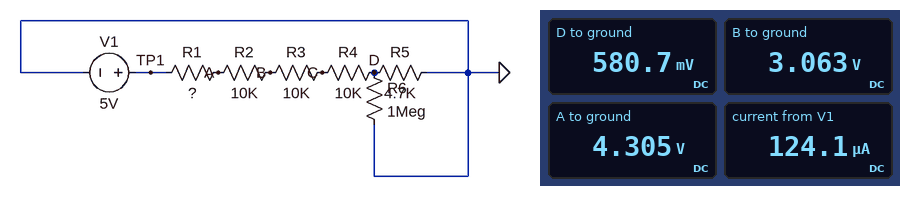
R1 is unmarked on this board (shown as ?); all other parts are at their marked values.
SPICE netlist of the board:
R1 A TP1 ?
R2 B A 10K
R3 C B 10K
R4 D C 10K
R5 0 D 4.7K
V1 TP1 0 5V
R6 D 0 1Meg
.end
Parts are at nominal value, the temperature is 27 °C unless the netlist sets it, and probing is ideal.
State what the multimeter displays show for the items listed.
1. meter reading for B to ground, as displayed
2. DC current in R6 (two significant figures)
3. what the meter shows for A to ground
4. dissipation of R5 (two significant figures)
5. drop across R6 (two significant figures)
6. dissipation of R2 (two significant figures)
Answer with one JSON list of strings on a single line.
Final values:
["3.063 V", "580 nA", "4.305 V", "72 µW", "580 mV", "150 µW"]
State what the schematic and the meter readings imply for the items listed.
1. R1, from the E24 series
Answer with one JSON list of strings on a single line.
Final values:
["5.6 kΩ"]
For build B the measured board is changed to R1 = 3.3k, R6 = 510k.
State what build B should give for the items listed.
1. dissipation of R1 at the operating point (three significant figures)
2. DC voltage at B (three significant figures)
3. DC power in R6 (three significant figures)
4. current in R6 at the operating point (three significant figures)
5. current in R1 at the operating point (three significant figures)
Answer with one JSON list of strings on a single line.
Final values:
["57.3 µW", "3.25 V", "738 nW", "1.20 µA", "132 µA"]
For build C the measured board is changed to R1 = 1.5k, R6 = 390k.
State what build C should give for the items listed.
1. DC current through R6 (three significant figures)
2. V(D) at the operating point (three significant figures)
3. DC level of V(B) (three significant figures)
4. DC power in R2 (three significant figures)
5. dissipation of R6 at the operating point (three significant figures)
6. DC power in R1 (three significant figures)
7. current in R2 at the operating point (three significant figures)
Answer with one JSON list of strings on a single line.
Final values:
["1.65 µA", "642 mV", "3.41 V", "191 µW", "1.06 µW", "28.7 µW", "138 µA"]
